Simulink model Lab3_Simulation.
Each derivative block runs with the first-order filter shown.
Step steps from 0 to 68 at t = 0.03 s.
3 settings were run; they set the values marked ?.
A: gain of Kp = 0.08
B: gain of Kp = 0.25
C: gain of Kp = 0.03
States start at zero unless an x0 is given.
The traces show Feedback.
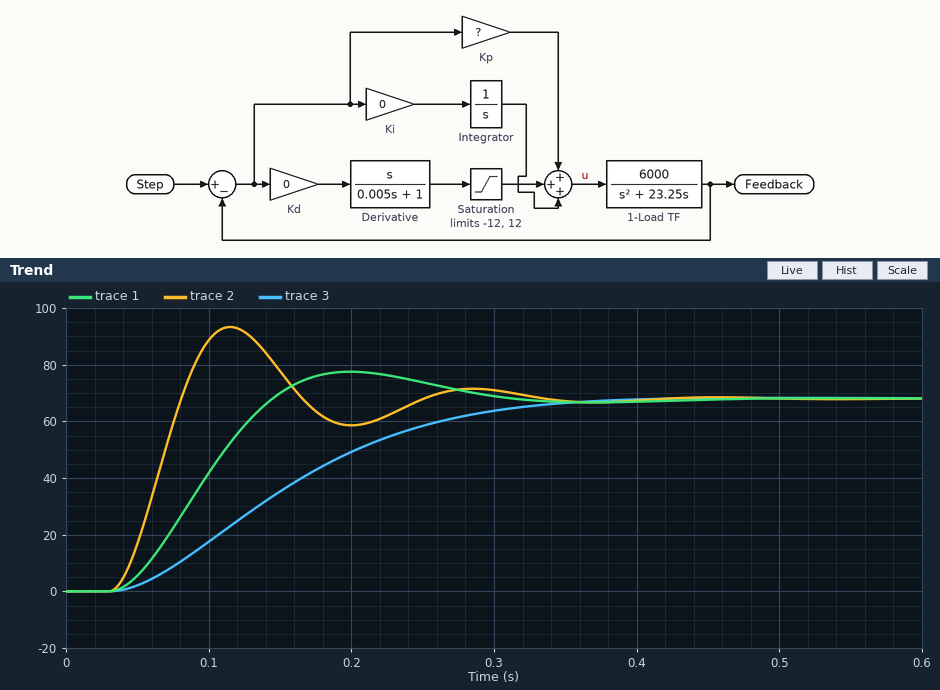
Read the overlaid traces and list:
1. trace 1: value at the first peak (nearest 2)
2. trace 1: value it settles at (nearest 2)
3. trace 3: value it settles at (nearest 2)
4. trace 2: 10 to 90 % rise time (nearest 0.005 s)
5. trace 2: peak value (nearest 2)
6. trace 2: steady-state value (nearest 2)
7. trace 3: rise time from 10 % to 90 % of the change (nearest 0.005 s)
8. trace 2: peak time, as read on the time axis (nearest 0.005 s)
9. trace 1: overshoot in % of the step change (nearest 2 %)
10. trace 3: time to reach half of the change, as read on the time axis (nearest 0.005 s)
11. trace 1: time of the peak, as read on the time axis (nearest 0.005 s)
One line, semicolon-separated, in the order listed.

78; 68; 68; 0.035 s; 94; 68; 0.205 s; 0.115 s; 14 %; 0.145 s; 0.200 s
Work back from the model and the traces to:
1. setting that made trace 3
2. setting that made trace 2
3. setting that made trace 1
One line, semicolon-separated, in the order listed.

C; B; A
